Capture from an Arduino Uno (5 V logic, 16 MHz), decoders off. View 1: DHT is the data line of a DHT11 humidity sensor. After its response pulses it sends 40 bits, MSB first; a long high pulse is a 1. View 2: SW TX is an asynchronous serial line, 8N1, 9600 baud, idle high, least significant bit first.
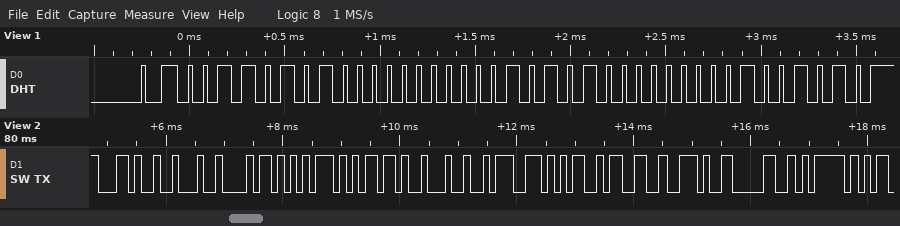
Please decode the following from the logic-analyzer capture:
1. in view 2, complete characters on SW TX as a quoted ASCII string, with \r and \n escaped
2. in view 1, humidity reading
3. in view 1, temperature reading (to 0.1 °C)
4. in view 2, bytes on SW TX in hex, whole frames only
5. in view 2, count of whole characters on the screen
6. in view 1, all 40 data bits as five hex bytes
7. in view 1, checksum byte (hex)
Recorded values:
",\"hum\":53.0}"
53 %
21.0 °C
0x2C 0x22 0x68 0x75 0x6D 0x22 0x3A 0x35 0x33 0x2E 0x30 0x7D
12
35 00 15 00 4A
0x4A
